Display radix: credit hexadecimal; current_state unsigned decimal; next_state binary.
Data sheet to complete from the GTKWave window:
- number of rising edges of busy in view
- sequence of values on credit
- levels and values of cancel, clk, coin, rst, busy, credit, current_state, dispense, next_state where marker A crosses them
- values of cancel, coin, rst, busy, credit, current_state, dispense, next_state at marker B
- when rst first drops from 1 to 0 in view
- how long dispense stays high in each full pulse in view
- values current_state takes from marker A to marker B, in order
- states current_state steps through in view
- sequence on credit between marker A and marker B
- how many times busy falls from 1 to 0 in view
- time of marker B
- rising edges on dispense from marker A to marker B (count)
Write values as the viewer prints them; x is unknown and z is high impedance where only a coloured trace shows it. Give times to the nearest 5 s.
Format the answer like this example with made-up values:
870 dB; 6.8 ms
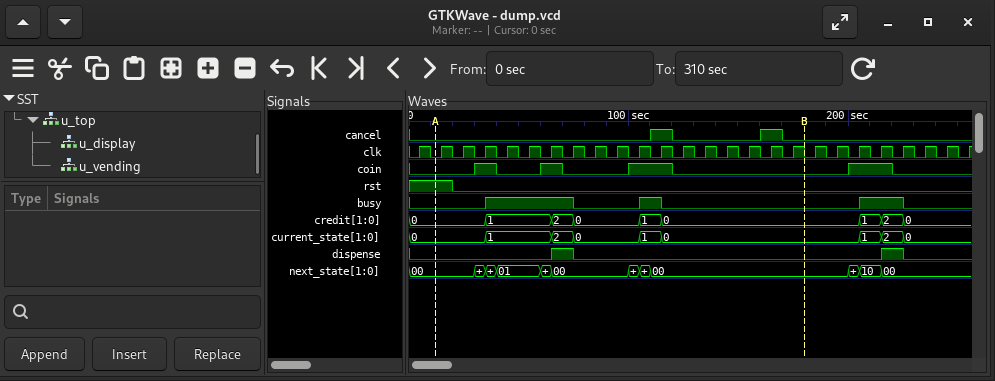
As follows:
3; 0, 1, 2, 0, 1, 0, 1, 2, 0; cancel=0, clk=0, coin=0, rst=1, busy=0, credit=0, current_state=0, dispense=0, next_state=00; cancel=0, coin=0, rst=0, busy=0, credit=0, current_state=0, dispense=0, next_state=00; 20 s; 10 s, 10 s; 0, 1, 2, 0, 1, 0; 0, 1, 2, 0, 1, 0, 1, 2, 0; 0, 1, 2, 0, 1, 0; 3; 180 s; 1
